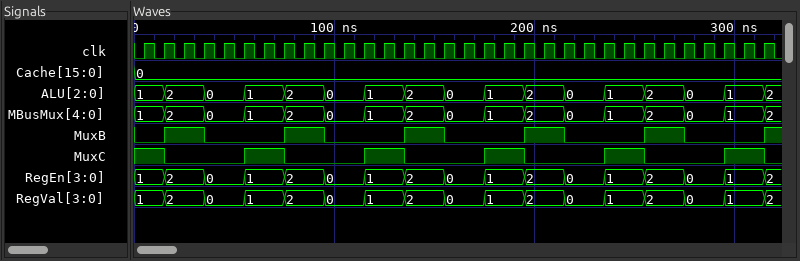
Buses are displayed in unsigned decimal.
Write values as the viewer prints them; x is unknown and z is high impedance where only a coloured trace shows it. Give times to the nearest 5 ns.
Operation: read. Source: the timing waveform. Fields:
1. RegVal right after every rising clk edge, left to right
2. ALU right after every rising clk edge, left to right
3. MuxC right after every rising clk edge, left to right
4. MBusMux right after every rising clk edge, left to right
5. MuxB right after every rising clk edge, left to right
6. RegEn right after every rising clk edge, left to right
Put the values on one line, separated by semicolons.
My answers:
1, 2, 2, 0, 0, 1, 1, 2, 2, 0, 0, 1, 1, 2, 2, 0, 0, 1, 1, 2, 2, 0, 0, 1, 1, 2, 2, 0, 0, 1, 1, 2; 1, 2, 2, 0, 0, 1, 1, 2, 2, 0, 0, 1, 1, 2, 2, 0, 0, 1, 1, 2, 2, 0, 0, 1, 1, 2, 2, 0, 0, 1, 1, 2; 1 0 0 0 0 1 1 0 0 0 0 1 1 0 0 0 0 1 1 0 0 0 0 1 1 0 0 0 0 1 1 0; 1, 2, 2, 0, 0, 1, 1, 2, 2, 0, 0, 1, 1, 2, 2, 0, 0, 1, 1, 2, 2, 0, 0, 1, 1, 2, 2, 0, 0, 1, 1, 2; 0 1 1 0 0 0 0 1 1 0 0 0 0 1 1 0 0 0 0 1 1 0 0 0 0 1 1 0 0 0 0 1; 1, 2, 2, 0, 0, 1, 1, 2, 2, 0, 0, 1, 1, 2, 2, 0, 0, 1, 1, 2, 2, 0, 0, 1, 1, 2, 2, 0, 0, 1, 1, 2
